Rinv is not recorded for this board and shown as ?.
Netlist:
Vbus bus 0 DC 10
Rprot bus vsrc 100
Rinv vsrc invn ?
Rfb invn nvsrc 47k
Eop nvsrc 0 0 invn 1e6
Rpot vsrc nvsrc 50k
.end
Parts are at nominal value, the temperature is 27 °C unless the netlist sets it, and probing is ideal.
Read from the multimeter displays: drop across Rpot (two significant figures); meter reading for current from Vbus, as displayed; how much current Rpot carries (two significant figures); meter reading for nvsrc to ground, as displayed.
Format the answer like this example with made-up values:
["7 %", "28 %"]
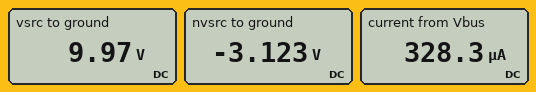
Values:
["13 V", "328.3 µA", "260 µA", "-3.123 V"]
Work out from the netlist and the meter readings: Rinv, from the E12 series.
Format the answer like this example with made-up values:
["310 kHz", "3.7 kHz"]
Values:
["150 kΩ"]
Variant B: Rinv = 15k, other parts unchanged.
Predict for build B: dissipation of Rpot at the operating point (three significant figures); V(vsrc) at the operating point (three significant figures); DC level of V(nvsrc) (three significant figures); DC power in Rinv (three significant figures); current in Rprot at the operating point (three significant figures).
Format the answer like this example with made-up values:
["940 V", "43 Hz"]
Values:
["33.2 mW", "9.85 V", "-30.9 V", "6.47 mW", "1.47 mA"]
